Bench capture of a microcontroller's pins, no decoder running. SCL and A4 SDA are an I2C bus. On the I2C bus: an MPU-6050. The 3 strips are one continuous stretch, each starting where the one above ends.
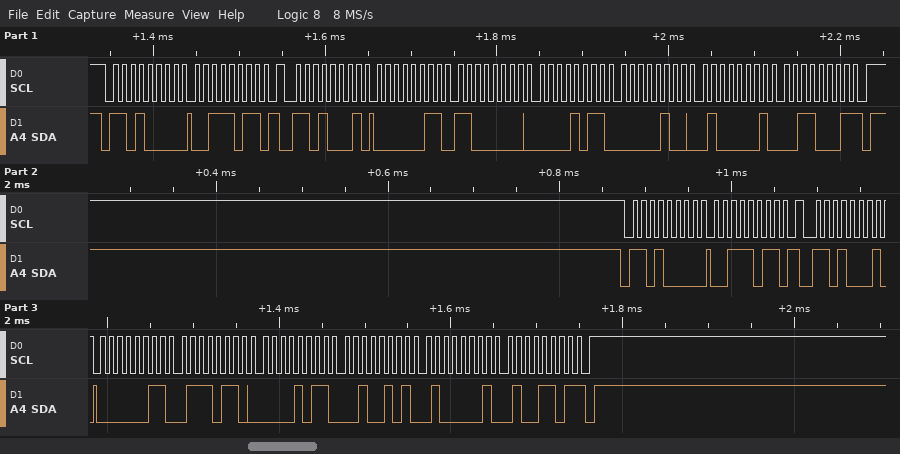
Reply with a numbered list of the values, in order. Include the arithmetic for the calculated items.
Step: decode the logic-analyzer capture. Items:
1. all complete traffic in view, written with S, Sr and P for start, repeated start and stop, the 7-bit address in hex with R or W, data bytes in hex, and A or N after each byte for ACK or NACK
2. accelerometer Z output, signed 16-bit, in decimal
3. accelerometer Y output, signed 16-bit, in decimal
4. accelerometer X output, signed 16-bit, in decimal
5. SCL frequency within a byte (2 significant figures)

1. S 68W A 3B A Sr 68R A 03 A C0 A 0B A 04 A 41 A 31 N P S 68W A 3B A Sr 68R A 03 A 76 A 0B A 25 A 41 A 4D N P
2. 0x4131 = 16689
3. 0x0B04 = 2820
4. 0x03C0 = 960
5. 100 kHz
